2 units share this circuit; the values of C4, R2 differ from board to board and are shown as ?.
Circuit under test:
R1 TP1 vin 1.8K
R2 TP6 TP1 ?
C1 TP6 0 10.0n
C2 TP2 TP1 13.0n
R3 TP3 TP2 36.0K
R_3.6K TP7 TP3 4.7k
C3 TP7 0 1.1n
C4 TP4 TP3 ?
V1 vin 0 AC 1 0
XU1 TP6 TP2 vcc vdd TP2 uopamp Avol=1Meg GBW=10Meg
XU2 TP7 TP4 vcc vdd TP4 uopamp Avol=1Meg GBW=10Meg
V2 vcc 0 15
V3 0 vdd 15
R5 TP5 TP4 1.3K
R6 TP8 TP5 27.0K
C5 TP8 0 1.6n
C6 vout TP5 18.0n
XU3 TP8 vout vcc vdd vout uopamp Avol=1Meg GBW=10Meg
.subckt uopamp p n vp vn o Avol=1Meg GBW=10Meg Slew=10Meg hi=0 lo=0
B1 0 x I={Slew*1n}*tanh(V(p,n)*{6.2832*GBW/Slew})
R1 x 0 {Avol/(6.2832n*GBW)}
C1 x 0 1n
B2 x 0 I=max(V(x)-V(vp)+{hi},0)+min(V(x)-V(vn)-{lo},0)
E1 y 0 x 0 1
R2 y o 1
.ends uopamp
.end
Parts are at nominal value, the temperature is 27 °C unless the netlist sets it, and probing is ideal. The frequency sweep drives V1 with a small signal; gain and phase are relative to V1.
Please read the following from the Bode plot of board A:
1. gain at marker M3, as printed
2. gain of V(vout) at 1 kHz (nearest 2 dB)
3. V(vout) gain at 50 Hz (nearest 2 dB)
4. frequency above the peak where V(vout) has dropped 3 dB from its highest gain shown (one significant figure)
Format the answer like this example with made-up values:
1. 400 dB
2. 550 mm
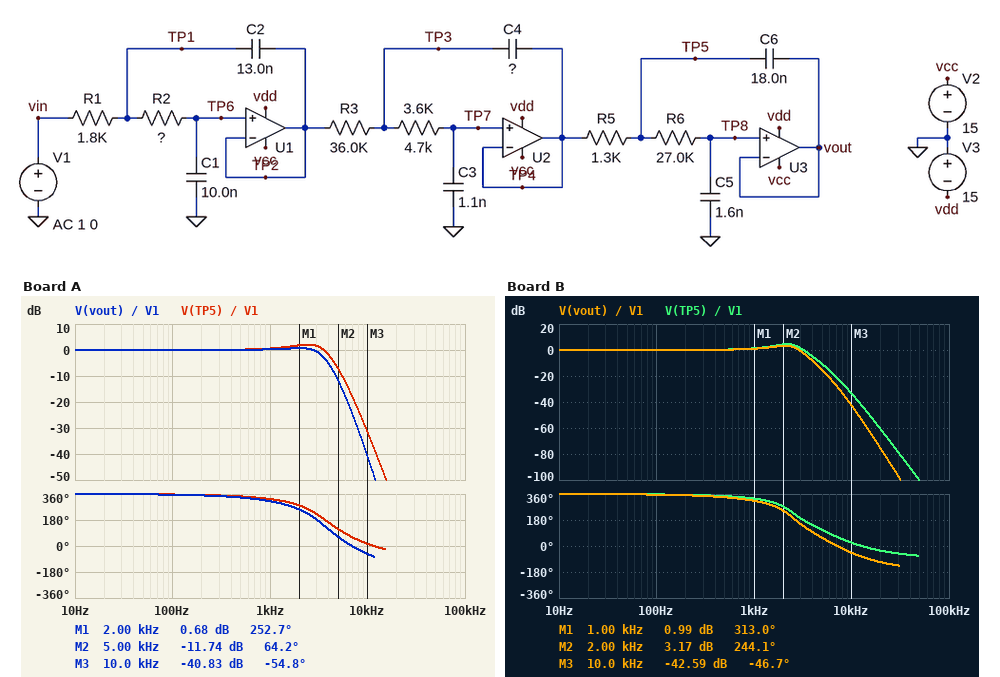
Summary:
1. -40.83 dB
2. 0 dB
3. 0 dB
4. 3 kHz
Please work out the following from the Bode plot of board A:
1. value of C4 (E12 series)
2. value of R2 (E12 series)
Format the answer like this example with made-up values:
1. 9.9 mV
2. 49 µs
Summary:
1. 12 nF
2. 2.7 kΩ
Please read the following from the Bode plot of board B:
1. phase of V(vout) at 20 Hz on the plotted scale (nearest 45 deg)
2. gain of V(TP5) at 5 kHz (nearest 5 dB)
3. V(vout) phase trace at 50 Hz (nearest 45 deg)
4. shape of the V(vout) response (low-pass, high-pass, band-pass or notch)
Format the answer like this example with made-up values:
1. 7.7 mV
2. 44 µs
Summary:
1. 360 deg
2. -10 dB
3. 360 deg
4. low-pass
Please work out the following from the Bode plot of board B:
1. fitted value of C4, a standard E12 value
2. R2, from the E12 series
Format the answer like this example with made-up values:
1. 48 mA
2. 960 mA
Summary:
1. 22 nF
2. 1.5 kΩ
